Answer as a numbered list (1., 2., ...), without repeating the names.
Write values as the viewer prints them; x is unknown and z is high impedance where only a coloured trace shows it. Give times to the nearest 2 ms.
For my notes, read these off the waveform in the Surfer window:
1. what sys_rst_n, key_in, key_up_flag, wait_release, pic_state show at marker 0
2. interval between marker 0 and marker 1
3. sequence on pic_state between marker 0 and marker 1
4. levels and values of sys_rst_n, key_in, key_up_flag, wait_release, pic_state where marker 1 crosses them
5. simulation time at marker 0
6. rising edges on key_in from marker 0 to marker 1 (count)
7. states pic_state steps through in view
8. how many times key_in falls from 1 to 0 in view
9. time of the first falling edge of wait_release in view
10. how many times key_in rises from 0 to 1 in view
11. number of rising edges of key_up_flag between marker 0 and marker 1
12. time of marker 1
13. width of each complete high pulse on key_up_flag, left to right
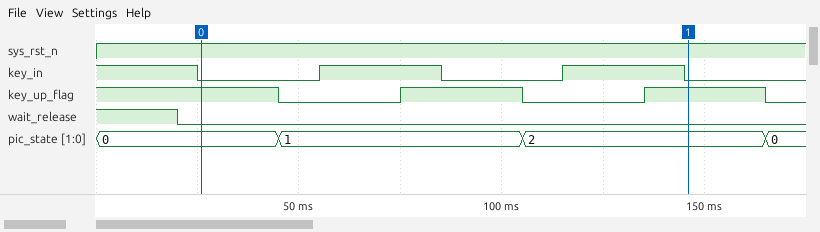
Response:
1. sys_rst_n=1, key_in=0, key_up_flag=1, wait_release=0, pic_state=0
2. 120 ms
3. 0, 1, 2
4. sys_rst_n=1, key_in=0, key_up_flag=1, wait_release=0, pic_state=2
5. 26 ms
6. 2
7. 0, 1, 2, 0
8. 3
9. 20 ms
10. 2
11. 2
12. 146 ms
13. 30 ms, 30 ms
